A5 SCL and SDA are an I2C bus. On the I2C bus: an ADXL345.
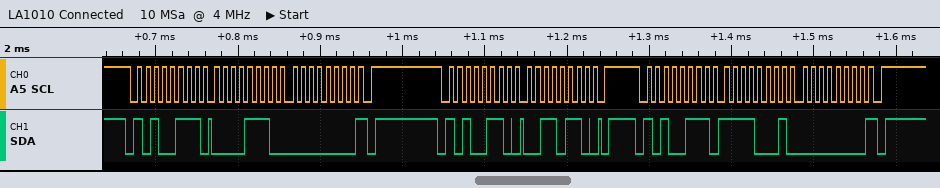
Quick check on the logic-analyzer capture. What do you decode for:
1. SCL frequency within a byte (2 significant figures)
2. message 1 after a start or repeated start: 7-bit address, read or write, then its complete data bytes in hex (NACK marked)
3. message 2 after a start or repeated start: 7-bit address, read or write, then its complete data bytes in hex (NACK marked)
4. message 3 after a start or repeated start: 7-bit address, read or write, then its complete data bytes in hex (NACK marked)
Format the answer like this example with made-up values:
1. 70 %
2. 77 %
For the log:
1. 100 kHz
2. 0x53 read: 0E 00 NACK
3. 0x53 write: 36
4. 0x53 read: F1 00 NACK
